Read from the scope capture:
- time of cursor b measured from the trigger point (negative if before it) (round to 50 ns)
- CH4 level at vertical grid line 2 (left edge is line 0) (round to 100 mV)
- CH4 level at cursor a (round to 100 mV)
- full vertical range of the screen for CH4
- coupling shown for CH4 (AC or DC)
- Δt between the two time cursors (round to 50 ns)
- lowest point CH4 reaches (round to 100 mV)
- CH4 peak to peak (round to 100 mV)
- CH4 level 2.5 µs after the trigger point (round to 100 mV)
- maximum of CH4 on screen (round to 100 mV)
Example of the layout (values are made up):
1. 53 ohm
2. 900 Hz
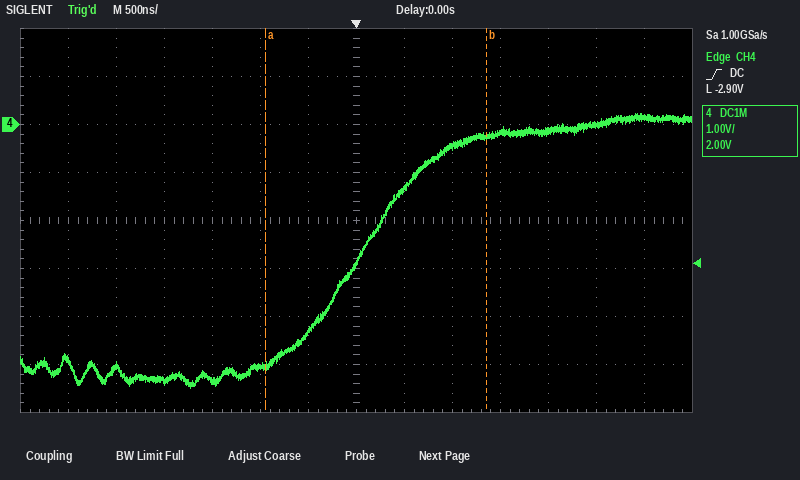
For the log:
1. +1.35 µs
2. -5.0 V
3. -5.0 V
4. 8 V
5. DC
6. 2.30 µs
7. -5.5 V
8. 5.7 V
9. 0.0 V
10. 200 mV
